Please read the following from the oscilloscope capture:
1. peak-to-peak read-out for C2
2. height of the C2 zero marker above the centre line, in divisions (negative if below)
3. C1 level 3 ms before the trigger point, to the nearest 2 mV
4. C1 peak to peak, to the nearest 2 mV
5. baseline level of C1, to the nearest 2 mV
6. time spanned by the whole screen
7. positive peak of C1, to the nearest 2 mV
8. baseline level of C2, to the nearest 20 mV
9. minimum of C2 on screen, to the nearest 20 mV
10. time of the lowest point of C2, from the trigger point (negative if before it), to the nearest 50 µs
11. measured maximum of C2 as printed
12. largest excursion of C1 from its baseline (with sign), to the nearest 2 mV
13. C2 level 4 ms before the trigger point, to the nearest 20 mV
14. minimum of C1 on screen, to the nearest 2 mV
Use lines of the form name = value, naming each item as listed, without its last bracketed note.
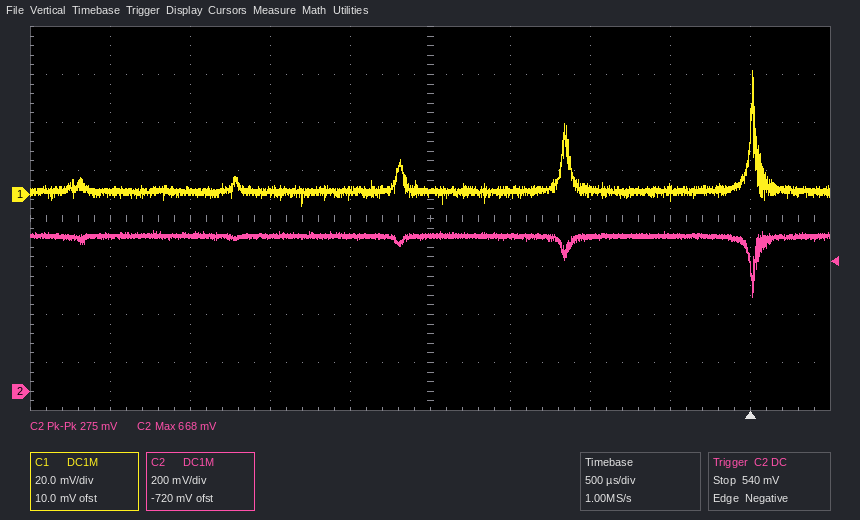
peak-to-peak read-out for C2 = 275 mV
height of the C2 zero marker above the centre line, in divisions = -3.6 div
C1 level 3 ms before the trigger point, to the nearest 2 mV = 2 mV
C1 peak to peak, to the nearest 2 mV = 56 mV
baseline level of C1, to the nearest 2 mV = 2 mV
time spanned by the whole screen = 5 ms
positive peak of C1, to the nearest 2 mV = 52 mV
baseline level of C2, to the nearest 20 mV = 640 mV
minimum of C2 on screen, to the nearest 20 mV = 400 mV
time of the lowest point of C2, from the trigger point (negative if before it), to the nearest 50 µs = 0 µs
measured maximum of C2 as printed = 668 mV
largest excursion of C1 from its baseline (with sign), to the nearest 2 mV = +50 mV
C2 level 4 ms before the trigger point, to the nearest 20 mV = 640 mV
minimum of C1 on screen, to the nearest 2 mV = -4 mV
